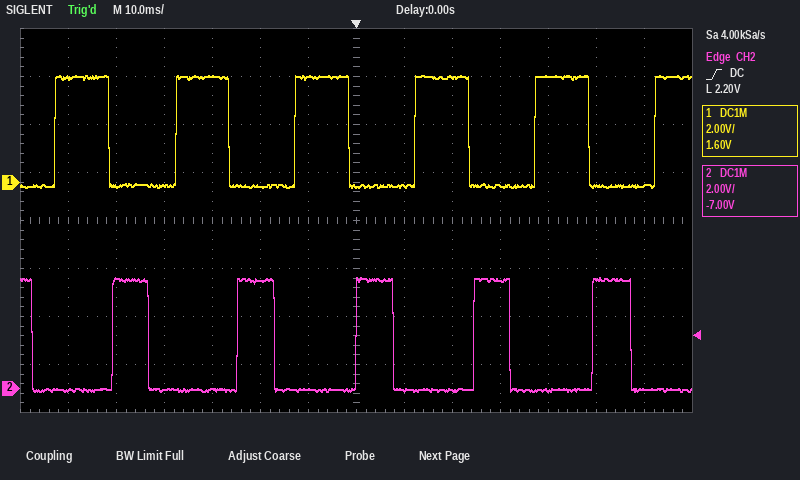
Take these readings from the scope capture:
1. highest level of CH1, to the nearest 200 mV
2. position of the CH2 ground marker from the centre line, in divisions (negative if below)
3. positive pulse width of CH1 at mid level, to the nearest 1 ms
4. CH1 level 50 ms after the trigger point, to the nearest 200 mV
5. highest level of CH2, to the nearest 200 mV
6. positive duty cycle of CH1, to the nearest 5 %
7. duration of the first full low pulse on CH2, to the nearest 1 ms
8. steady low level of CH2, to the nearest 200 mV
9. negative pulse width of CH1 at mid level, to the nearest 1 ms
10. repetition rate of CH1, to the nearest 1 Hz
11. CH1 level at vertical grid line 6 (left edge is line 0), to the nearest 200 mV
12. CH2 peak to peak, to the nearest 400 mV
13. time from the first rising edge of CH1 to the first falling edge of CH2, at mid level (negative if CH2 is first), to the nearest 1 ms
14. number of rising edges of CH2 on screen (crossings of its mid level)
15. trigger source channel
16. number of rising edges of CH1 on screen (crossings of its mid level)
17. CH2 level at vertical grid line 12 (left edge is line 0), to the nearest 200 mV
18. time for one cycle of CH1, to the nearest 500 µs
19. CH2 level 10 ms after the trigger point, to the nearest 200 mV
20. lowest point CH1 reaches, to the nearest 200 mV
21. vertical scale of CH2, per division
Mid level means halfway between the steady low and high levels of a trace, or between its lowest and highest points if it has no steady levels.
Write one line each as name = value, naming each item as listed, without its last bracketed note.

highest level of CH1, to the nearest 200 mV = 4.4 V
position of the CH2 ground marker from the centre line, in divisions = -3.5 div
positive pulse width of CH1 at mid level, to the nearest 1 ms = 11 ms
CH1 level 50 ms after the trigger point, to the nearest 200 mV = -200 mV
highest level of CH2, to the nearest 200 mV = 4.6 V
positive duty cycle of CH1, to the nearest 5 % = 45 %
duration of the first full low pulse on CH2, to the nearest 1 ms = 17 ms
steady low level of CH2, to the nearest 200 mV = 0.0 V
negative pulse width of CH1 at mid level, to the nearest 1 ms = 14 ms
repetition rate of CH1, to the nearest 1 Hz = 40 Hz
CH1 level at vertical grid line 6 (left edge is line 0), to the nearest 200 mV = 4.4 V
CH2 peak to peak, to the nearest 400 mV = 4.8 V
time from the first rising edge of CH1 to the first falling edge of CH2, at mid level (negative if CH2 is first), to the nearest 1 ms = -5 ms
number of rising edges of CH2 on screen = 5
trigger source channel = CH2
number of rising edges of CH1 on screen = 6
CH2 level at vertical grid line 12 (left edge is line 0), to the nearest 200 mV = 4.6 V
time for one cycle of CH1, to the nearest 500 µs = 25.0 ms
CH2 level 10 ms after the trigger point, to the nearest 200 mV = 0.0 V
lowest point CH1 reaches, to the nearest 200 mV = -200 mV
vertical scale of CH2, per division = 2 V
